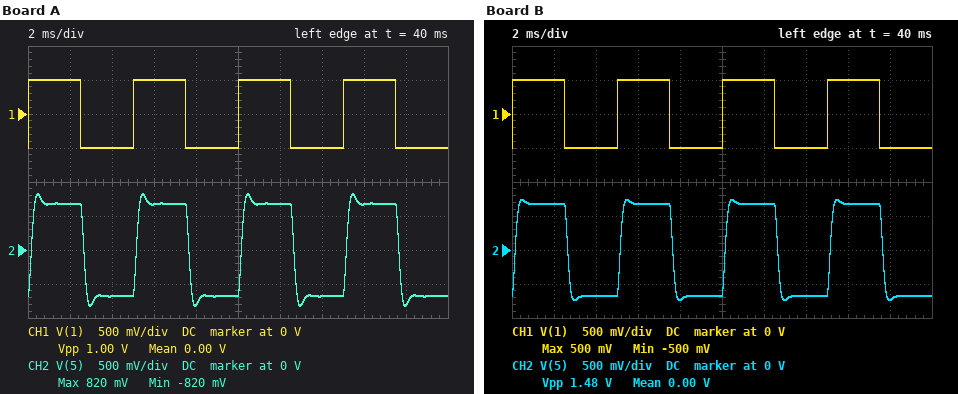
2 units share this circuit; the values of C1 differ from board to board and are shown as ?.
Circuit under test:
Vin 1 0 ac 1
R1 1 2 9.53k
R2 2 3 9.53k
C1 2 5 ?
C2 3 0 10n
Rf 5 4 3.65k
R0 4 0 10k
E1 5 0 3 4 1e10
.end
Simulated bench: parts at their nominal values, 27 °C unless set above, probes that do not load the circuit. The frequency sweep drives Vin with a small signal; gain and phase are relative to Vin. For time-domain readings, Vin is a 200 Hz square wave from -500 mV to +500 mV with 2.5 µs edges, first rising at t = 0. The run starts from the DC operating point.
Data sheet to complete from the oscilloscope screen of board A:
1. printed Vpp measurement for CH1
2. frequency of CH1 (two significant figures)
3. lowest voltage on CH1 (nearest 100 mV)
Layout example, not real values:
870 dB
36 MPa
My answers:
1.00 V
200 Hz
-500 mV
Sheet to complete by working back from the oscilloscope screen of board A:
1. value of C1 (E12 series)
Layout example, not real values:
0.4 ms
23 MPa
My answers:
15 nF
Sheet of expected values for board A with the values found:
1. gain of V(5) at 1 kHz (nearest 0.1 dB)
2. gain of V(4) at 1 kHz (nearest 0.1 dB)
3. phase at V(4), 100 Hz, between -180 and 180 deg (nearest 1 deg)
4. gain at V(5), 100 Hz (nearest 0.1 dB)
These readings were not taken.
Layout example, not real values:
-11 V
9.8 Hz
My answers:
2.8 dB
0.1 dB
-5 deg
2.7 dB
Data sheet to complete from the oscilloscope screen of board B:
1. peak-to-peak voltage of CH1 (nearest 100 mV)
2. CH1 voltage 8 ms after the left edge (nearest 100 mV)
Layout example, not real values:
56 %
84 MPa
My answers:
1.0 V
-500 mV
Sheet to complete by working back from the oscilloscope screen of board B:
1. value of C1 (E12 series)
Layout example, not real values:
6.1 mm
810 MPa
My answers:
12 nF
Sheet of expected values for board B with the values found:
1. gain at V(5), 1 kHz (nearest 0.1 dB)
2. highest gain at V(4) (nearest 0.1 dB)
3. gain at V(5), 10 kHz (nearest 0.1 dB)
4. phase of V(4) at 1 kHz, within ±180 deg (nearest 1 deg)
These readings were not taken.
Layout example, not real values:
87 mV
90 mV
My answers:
1.9 dB
0 dB
-30.0 dB
-59 deg
